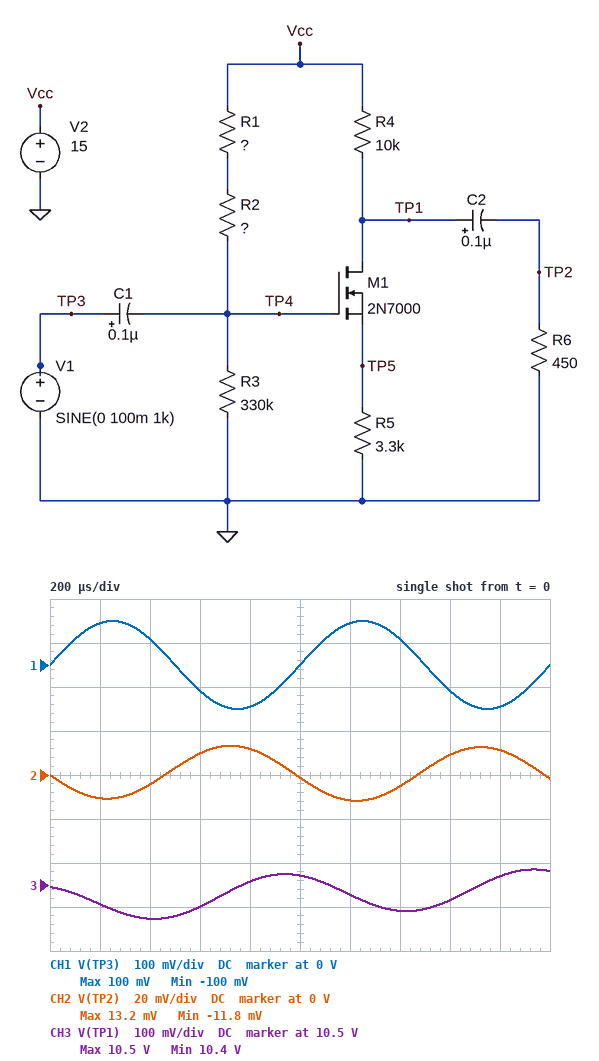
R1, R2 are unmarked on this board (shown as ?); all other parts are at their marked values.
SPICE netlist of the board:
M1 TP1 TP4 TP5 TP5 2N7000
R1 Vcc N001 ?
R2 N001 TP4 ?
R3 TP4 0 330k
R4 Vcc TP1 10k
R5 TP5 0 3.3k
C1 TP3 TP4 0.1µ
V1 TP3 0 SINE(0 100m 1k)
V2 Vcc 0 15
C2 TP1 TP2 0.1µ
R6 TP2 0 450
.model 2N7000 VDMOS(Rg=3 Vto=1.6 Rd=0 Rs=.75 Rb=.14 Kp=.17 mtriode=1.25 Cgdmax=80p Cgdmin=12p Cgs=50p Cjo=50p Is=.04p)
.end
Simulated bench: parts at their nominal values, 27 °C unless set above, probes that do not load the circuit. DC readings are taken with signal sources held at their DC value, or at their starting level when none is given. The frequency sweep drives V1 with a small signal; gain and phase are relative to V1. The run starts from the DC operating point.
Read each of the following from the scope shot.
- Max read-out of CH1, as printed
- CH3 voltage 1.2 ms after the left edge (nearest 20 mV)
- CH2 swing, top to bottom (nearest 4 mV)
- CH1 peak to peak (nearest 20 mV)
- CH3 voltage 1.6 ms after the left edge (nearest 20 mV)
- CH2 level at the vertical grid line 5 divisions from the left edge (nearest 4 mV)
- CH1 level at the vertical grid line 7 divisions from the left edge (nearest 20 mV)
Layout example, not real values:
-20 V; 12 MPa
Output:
100 mV; 10.48 V; 24 mV; 200 mV; 10.46 V; 0 V; 60 mV
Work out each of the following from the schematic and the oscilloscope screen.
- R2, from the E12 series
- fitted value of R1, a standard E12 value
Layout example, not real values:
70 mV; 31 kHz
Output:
270 kΩ; 1 MΩ
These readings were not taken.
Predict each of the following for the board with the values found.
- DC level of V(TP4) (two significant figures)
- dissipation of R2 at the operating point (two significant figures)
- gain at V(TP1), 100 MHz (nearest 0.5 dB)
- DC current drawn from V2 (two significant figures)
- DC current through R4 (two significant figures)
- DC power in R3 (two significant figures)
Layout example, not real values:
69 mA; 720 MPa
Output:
3.1 V; 24 µW; 0 dB; 460 µA; 450 µA; 29 µW
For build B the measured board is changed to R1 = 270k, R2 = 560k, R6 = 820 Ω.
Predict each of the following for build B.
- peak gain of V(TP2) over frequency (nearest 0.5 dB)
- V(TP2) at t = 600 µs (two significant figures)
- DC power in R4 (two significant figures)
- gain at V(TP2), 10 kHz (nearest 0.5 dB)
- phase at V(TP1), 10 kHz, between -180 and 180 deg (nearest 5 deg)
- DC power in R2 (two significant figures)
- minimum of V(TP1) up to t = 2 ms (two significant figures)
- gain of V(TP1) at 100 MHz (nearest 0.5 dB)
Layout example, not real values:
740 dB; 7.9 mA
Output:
0.5 dB; 17 mV; 6.3 mW; -13.0 dB; 170 deg; 94 µW; 7.0 V; 0 dB
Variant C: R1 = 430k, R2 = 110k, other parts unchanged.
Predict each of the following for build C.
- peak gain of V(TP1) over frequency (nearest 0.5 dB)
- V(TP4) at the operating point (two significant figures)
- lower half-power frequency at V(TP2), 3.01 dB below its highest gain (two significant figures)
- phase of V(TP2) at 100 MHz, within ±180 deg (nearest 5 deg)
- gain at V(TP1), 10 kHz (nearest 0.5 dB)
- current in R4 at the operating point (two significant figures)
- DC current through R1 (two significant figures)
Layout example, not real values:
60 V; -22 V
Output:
0 dB; 5.7 V; 3.3 MHz; 0 deg; -45.0 dB; 1.1 mA; 17 µA
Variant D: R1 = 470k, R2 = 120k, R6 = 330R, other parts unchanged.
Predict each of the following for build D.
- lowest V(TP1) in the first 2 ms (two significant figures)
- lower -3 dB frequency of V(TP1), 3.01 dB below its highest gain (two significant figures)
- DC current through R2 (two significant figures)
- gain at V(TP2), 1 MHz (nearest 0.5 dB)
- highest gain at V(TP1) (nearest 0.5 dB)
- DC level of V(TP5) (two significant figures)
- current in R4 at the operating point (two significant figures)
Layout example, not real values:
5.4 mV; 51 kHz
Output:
3.8 V; 7.1 Hz; 16 µA; -14.5 dB; 3.0 dB; 3.7 V; 1.1 mA
